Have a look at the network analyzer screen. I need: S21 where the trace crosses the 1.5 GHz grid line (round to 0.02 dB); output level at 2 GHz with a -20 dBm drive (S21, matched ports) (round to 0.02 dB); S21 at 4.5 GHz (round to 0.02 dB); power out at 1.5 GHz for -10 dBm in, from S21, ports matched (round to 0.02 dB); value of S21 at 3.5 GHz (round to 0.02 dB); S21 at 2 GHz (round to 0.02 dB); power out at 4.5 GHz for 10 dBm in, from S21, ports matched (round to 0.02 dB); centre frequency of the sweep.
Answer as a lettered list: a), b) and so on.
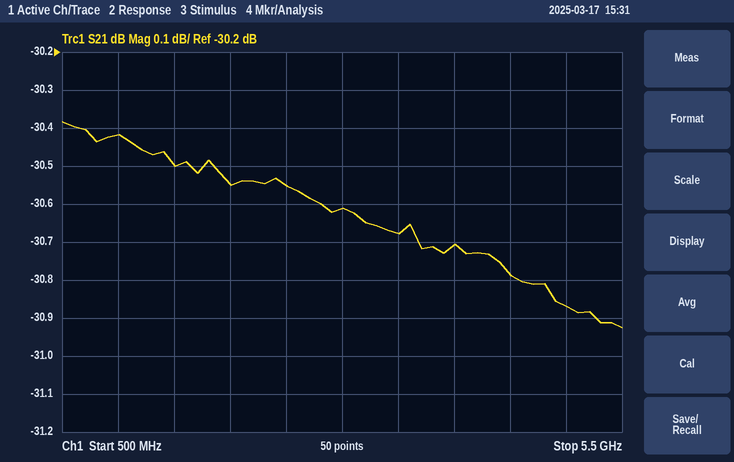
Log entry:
a) -30.50 dB
b) -50.54 dBm
c) -30.78 dB
d) -40.50 dBm
e) -30.68 dB
f) -30.54 dB
g) -20.78 dBm
h) 3 GHz
